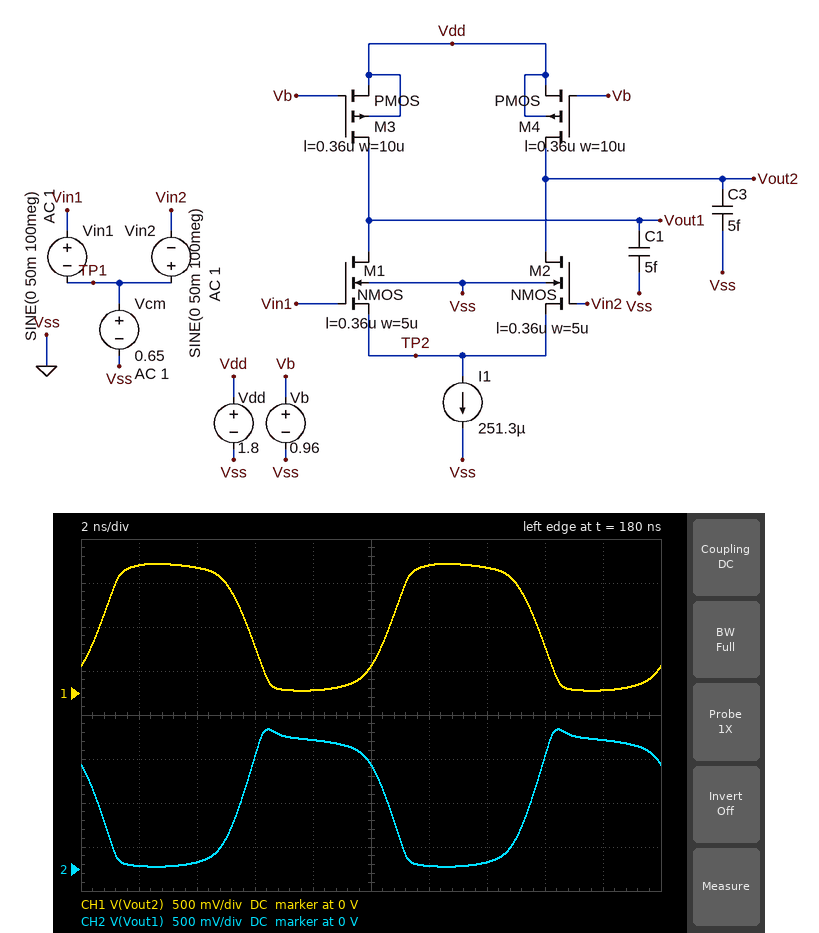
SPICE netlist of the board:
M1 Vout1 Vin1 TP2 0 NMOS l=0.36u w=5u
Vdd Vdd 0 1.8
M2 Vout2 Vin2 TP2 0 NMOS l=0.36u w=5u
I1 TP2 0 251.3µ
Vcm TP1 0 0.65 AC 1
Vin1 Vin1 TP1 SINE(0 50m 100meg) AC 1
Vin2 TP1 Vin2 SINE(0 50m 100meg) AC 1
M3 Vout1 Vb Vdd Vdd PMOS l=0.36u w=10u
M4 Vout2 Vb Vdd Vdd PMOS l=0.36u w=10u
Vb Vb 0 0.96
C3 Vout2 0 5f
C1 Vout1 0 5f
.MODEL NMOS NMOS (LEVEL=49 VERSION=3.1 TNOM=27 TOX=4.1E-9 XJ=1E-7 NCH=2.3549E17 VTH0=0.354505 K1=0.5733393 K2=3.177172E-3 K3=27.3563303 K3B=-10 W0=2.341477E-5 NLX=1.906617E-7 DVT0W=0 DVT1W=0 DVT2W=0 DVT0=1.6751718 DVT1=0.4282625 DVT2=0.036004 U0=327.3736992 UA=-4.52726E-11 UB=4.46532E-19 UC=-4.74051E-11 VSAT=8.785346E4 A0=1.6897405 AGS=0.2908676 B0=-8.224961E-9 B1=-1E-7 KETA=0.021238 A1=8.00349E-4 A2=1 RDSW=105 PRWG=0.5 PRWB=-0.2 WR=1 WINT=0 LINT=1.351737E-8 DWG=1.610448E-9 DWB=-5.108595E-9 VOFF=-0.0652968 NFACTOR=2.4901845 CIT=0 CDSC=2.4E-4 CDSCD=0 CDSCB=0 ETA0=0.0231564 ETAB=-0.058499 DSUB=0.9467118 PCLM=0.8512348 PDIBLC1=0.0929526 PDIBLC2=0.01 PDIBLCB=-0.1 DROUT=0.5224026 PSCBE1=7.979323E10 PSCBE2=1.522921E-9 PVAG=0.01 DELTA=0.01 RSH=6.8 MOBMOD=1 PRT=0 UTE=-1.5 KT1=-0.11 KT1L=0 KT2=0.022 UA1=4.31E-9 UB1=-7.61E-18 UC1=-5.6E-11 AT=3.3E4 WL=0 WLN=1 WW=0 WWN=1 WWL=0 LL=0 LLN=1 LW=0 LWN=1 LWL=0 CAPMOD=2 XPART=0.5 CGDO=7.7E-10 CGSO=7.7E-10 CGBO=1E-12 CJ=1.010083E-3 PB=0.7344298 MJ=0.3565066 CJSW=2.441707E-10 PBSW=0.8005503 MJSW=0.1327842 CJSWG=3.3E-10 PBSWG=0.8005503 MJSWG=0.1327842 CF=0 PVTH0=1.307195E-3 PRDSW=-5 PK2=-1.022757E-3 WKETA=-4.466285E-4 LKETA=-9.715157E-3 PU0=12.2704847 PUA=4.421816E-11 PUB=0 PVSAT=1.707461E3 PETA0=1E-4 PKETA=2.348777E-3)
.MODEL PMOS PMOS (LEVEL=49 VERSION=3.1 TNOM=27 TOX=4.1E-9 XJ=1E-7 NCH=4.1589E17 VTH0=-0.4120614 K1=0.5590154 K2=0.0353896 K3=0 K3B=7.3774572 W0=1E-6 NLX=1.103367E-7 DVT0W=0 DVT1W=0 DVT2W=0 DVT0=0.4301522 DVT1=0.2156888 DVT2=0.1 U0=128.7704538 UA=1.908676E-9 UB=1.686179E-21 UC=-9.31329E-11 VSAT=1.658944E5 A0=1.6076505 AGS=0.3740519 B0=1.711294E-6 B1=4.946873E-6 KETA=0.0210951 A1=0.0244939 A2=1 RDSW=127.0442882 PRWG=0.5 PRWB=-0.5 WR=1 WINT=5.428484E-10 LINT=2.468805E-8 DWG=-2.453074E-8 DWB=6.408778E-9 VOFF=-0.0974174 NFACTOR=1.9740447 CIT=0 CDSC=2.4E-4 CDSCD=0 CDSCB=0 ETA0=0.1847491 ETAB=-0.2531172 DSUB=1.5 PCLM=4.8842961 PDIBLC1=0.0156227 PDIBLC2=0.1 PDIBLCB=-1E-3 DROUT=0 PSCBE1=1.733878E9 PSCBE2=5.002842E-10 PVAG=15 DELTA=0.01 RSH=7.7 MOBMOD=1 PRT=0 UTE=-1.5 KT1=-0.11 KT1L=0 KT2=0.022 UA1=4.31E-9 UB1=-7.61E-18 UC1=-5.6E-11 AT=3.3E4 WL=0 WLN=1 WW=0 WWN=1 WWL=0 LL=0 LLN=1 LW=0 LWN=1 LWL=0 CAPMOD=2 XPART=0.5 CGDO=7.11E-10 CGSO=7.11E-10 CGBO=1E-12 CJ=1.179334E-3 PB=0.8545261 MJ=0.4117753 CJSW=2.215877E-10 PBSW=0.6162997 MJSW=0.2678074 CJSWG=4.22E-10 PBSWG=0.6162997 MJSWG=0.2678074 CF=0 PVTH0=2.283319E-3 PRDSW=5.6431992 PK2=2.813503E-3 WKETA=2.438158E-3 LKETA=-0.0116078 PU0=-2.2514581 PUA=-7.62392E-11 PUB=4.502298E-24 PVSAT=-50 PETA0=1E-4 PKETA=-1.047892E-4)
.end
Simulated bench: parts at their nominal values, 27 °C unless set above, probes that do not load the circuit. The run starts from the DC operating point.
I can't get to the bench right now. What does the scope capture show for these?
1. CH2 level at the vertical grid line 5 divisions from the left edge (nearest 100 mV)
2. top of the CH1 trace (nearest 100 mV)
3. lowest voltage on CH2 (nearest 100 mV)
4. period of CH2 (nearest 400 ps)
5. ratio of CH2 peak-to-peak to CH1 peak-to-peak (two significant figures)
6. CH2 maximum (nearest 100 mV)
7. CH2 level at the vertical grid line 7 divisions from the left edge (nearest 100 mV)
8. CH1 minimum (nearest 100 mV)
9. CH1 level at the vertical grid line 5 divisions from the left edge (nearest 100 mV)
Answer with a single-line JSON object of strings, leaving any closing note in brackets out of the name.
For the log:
{"CH2 level at the vertical grid line 5 divisions from the left edge": "1.2 V", "top of the CH1 trace": "1.5 V", "lowest voltage on CH2": "0 V", "period of CH2": "10.0 ns", "ratio of CH2 peak-to-peak to CH1 peak-to-peak": "1.1", "CH2 maximum": "1.6 V", "CH2 level at the vertical grid line 7 divisions from the left edge": "100 mV", "CH1 minimum": "0 V", "CH1 level at the vertical grid line 5 divisions from the left edge": "300 mV"}
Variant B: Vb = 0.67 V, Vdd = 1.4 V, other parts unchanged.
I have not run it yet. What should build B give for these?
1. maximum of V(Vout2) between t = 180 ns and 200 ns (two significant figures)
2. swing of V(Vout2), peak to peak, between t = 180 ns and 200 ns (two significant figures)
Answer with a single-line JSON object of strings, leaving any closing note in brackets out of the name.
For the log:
{"maximum of V(Vout2) between t = 180 ns and 200 ns": "-680 mV", "swing of V(Vout2), peak to peak, between t = 180 ns and 200 ns": "3.0 mV"}
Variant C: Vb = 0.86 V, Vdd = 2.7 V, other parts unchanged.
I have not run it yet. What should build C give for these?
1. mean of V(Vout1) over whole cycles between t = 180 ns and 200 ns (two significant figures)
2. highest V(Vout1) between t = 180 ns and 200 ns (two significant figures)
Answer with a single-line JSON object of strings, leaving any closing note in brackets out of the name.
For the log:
{"mean of V(Vout1) over whole cycles between t = 180 ns and 200 ns": "2.6 V", "highest V(Vout1) between t = 180 ns and 200 ns": "2.7 V"}
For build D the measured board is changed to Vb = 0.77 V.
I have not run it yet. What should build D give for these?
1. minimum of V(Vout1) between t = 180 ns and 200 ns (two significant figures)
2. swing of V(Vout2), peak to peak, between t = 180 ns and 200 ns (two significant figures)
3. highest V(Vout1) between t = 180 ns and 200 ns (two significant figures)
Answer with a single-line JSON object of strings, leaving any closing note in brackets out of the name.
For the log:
{"minimum of V(Vout1) between t = 180 ns and 200 ns": "1.6 V", "swing of V(Vout2), peak to peak, between t = 180 ns and 200 ns": "120 mV", "highest V(Vout1) between t = 180 ns and 200 ns": "1.7 V"}
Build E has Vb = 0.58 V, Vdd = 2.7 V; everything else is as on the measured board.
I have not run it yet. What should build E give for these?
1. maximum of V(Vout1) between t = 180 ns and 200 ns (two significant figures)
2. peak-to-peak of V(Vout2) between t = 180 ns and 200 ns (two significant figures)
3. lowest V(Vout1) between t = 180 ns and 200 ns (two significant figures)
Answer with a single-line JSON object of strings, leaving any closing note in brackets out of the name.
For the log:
{"maximum of V(Vout1) between t = 180 ns and 200 ns": "2.7 V", "peak-to-peak of V(Vout2) between t = 180 ns and 200 ns": "40 mV", "lowest V(Vout1) between t = 180 ns and 200 ns": "2.6 V"}
